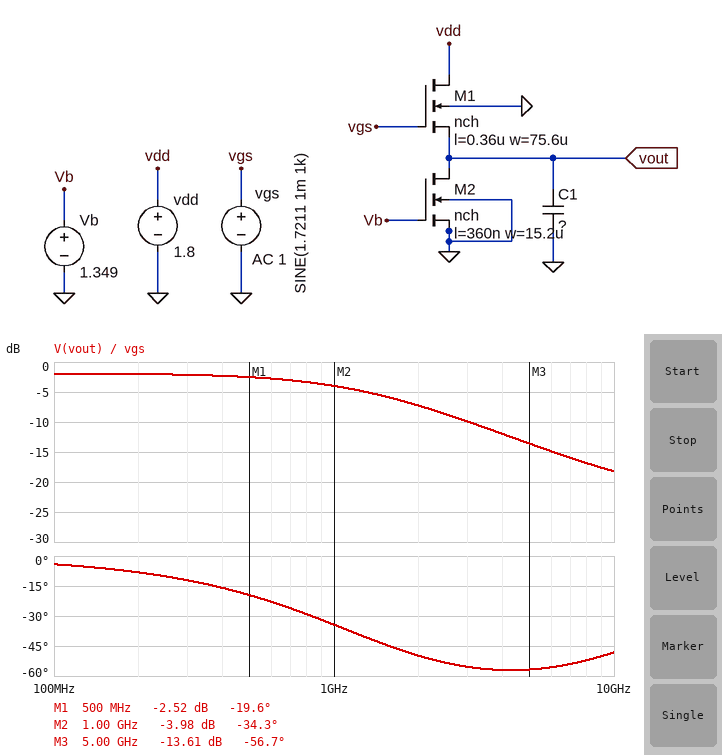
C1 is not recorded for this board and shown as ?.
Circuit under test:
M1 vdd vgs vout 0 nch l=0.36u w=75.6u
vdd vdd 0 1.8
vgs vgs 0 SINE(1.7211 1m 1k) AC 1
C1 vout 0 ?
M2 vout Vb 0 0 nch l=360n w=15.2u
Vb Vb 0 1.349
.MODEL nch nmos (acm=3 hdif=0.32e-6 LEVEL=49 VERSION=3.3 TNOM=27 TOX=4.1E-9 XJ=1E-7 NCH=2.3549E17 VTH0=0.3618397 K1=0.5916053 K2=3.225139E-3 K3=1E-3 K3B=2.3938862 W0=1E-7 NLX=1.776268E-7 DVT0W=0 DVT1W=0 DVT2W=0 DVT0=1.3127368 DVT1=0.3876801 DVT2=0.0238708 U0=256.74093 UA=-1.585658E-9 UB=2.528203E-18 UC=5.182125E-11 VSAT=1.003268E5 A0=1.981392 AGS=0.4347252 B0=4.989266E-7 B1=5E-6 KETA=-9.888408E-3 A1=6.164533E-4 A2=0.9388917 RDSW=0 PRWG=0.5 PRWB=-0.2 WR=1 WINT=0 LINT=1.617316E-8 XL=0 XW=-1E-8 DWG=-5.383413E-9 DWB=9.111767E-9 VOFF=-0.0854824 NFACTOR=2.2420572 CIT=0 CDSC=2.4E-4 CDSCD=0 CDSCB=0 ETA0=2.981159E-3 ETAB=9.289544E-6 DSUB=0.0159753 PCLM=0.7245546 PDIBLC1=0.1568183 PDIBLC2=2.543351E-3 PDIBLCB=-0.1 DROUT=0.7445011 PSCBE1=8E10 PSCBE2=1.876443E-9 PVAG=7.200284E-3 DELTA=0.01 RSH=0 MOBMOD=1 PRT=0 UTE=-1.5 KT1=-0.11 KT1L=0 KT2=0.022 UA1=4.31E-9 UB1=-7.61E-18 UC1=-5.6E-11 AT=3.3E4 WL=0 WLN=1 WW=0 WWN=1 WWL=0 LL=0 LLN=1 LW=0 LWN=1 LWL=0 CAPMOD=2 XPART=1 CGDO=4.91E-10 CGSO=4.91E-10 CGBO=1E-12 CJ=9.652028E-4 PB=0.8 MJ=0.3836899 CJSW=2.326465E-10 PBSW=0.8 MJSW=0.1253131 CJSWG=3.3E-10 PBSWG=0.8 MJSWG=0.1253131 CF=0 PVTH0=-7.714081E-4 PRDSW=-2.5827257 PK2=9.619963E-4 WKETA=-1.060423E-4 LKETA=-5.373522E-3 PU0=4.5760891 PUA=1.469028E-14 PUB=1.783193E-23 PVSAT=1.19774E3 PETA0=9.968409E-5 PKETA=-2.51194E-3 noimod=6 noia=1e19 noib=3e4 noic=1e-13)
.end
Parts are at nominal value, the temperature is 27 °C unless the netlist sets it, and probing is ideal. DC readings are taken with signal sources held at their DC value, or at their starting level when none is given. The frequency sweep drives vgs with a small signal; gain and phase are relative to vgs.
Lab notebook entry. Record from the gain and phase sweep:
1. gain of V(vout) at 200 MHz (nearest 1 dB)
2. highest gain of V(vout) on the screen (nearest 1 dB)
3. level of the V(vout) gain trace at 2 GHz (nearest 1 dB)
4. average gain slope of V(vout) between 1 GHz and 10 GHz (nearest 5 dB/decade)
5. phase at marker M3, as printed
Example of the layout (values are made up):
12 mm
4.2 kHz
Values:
-2 dB
-2 dB
-7 dB
-15 dB/decade
-56.7 deg
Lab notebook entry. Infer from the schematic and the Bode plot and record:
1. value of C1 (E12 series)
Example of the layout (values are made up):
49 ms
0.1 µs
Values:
2.2 pF
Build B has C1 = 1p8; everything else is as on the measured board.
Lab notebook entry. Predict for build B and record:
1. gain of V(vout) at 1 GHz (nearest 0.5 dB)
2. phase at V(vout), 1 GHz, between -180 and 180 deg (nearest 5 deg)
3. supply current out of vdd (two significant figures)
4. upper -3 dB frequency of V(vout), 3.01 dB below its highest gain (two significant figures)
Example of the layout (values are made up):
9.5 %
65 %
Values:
-3.5 dB
-30 deg
3.0 mA
1.5 GHz
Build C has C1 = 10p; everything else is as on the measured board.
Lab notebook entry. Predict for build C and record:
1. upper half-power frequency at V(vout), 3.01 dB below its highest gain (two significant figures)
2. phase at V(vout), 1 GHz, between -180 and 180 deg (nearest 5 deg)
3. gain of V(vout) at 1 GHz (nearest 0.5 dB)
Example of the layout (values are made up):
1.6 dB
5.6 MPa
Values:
310 MHz
-70 deg
-12.5 dB
